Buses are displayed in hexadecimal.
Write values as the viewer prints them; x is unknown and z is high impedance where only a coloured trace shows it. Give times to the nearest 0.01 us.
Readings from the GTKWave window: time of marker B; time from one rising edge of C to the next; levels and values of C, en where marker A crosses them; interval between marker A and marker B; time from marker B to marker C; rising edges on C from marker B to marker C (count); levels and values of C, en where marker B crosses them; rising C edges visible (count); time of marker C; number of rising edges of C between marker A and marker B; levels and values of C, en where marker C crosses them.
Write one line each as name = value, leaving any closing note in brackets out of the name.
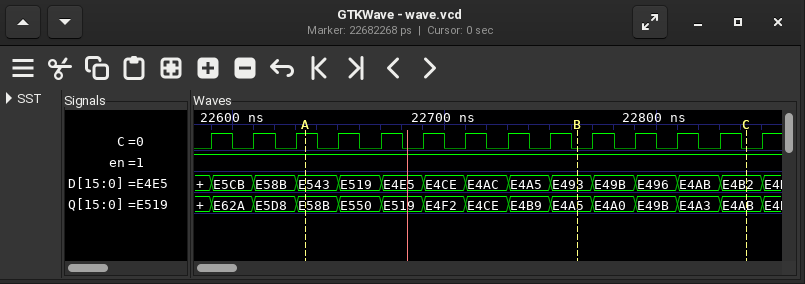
time of marker B = 22.76 us
time from one rising edge of C to the next = 0.02 us
levels and values of C, en where marker A crosses them = C=1, en=1
interval between marker A and marker B = 0.13 us
time from marker B to marker C = 0.08 us
rising edges on C from marker B to marker C = 4
levels and values of C, en where marker B crosses them = C=0, en=1
rising C edges visible = 14
time of marker C = 22.84 us
number of rising edges of C between marker A and marker B = 6
levels and values of C, en where marker C crosses them = C=0, en=1
